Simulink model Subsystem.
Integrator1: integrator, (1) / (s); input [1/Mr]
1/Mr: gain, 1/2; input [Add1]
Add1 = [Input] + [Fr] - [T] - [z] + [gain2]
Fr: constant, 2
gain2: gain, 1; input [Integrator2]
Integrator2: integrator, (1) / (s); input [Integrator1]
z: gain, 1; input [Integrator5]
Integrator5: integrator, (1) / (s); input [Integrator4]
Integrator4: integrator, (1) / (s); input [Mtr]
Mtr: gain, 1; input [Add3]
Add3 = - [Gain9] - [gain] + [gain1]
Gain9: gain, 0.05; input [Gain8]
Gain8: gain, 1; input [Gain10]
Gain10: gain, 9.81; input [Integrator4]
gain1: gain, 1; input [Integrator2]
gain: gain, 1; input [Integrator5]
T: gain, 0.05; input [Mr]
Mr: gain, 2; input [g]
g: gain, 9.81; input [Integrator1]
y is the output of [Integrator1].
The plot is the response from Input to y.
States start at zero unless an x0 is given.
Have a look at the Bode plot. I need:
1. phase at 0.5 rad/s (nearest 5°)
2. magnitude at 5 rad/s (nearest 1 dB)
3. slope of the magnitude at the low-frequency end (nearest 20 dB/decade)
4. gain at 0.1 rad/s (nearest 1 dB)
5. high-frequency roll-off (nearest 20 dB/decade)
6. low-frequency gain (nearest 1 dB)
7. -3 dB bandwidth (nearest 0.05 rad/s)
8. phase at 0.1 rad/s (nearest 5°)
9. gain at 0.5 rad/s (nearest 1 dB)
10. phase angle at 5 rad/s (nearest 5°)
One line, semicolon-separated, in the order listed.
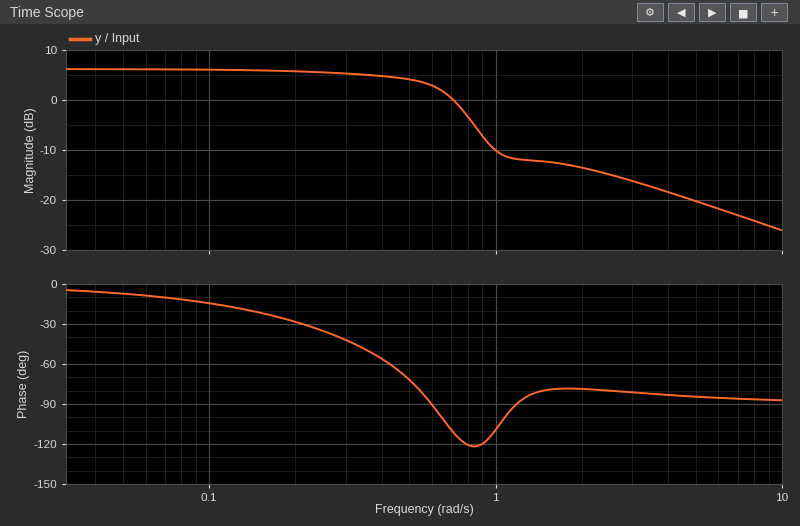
-70°; -20 dB; 0 dB/decade; 6 dB; -20 dB/decade; 6 dB; 0.60 rad/s; -15°; 4 dB; -85°
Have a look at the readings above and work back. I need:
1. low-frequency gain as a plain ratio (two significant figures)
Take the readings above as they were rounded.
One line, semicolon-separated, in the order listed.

2.0
